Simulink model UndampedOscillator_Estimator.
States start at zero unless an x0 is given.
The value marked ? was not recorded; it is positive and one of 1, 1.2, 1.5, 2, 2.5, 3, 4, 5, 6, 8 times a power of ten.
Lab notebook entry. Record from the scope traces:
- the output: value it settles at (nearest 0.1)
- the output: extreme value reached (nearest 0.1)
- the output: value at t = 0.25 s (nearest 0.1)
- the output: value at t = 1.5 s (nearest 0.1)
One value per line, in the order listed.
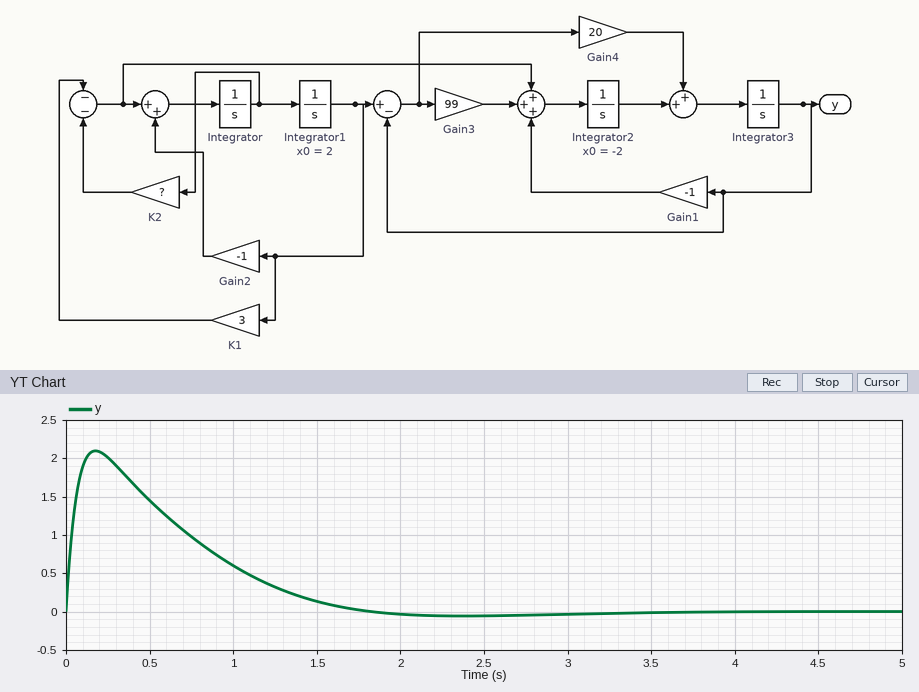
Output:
0.0
2.1
2.0
0.1
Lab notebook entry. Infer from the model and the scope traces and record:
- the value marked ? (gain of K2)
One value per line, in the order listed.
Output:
3
